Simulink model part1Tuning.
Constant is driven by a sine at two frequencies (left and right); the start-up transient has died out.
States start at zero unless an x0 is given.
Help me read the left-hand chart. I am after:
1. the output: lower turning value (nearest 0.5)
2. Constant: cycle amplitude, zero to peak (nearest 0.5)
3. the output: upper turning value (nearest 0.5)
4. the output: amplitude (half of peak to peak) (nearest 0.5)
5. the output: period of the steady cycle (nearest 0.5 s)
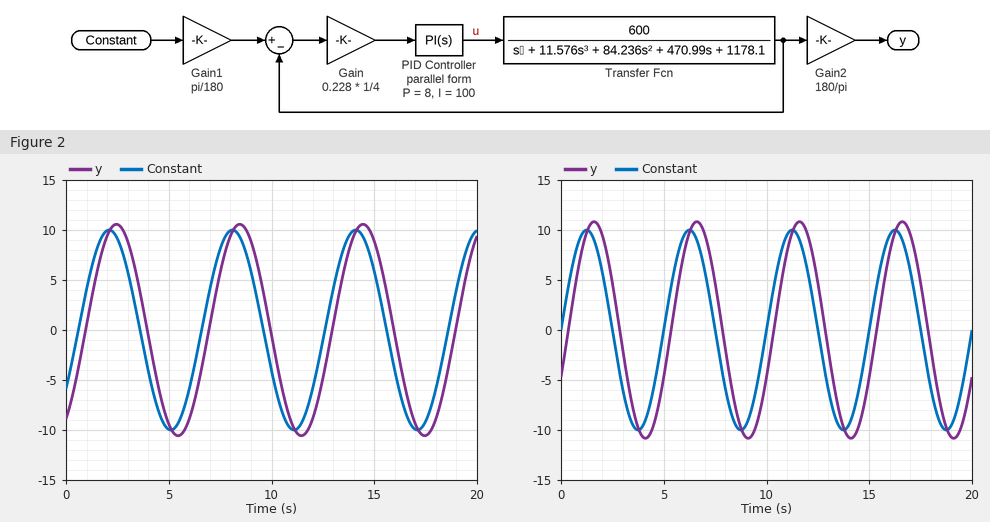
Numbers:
-10.5
10.0
10.5
10.5
6.0 s
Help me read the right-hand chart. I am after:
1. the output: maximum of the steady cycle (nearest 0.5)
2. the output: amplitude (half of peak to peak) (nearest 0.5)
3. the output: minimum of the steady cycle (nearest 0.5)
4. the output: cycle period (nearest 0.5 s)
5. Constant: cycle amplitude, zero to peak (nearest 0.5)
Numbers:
11.0
11.0
-11.0
5.0 s
10.0
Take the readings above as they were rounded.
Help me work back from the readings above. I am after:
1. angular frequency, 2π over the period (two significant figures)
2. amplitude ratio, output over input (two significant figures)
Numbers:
1.3 rad/s
1.1
